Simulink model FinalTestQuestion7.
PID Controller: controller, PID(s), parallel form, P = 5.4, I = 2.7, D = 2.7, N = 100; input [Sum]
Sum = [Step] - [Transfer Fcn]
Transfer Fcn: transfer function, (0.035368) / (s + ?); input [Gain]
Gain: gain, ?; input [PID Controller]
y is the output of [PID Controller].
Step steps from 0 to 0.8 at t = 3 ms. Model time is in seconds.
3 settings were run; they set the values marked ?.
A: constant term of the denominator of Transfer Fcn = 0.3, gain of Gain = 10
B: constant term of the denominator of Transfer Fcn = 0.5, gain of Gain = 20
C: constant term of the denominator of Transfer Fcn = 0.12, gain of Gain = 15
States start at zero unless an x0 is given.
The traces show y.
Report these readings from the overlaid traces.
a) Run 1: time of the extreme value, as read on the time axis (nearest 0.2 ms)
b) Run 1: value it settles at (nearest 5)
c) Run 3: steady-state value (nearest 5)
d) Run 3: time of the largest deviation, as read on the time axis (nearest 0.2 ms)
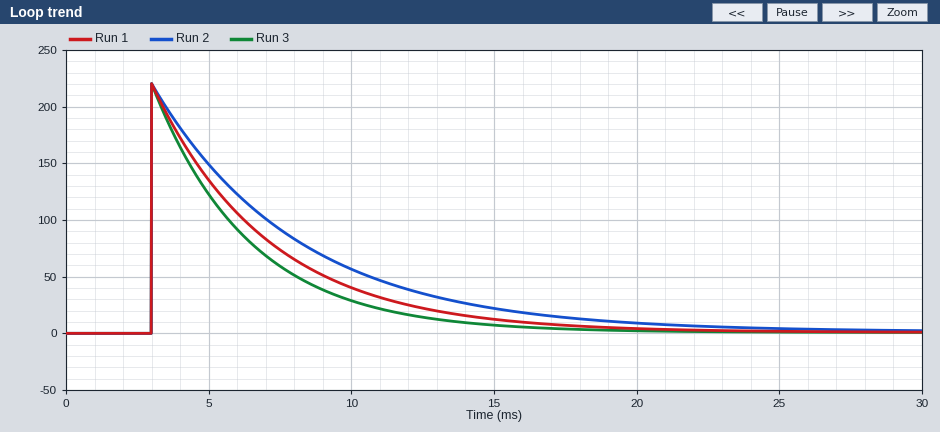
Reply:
3.0 ms
0
0
3.0 ms
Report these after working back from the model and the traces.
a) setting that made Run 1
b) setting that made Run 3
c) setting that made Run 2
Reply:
C
B
A
